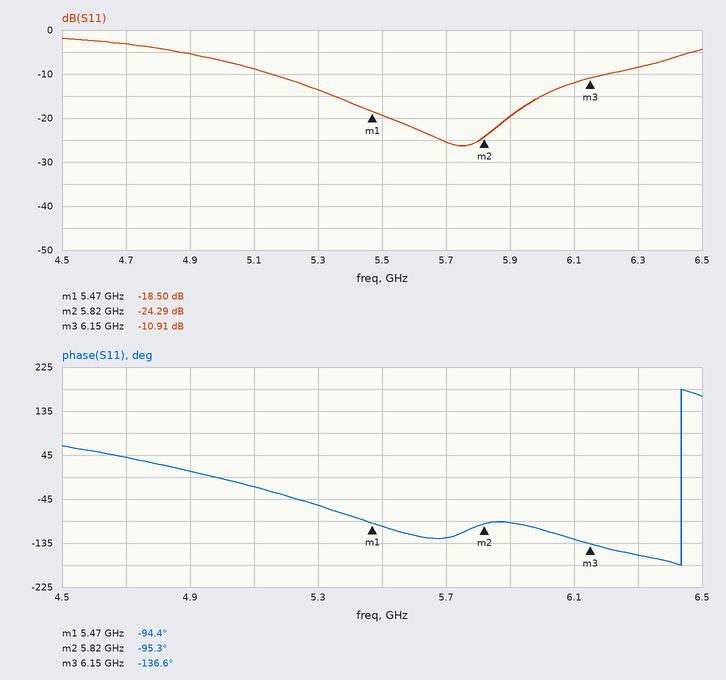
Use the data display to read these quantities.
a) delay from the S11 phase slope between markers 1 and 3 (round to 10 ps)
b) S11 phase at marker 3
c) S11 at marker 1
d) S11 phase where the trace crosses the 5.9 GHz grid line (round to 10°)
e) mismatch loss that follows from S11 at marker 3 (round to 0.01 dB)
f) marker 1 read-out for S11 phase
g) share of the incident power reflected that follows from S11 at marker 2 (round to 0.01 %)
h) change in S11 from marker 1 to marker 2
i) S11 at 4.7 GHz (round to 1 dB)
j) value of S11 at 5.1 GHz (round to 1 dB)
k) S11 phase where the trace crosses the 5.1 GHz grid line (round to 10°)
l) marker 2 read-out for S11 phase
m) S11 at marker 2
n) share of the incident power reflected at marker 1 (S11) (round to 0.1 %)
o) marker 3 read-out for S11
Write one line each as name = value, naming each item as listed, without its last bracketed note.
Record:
delay from the S11 phase slope between markers 1 and 3 = 170 ps
S11 phase at marker 3 = -136.6°
S11 at marker 1 = -18.50 dB
S11 phase where the trace crosses the 5.9 GHz grid line = -90°
mismatch loss that follows from S11 at marker 3 = 0.37 dB
marker 1 read-out for S11 phase = -94.4°
share of the incident power reflected that follows from S11 at marker 2 = 0.37 %
change in S11 from marker 1 to marker 2 = -5.79 dB
S11 at 4.7 GHz = -3 dB
value of S11 at 5.1 GHz = -9 dB
S11 phase where the trace crosses the 5.1 GHz grid line = -20°
marker 2 read-out for S11 phase = -95.3°
S11 at marker 2 = -24.29 dB
share of the incident power reflected at marker 1 (S11) = 1.4 %
marker 3 read-out for S11 = -10.91 dB
